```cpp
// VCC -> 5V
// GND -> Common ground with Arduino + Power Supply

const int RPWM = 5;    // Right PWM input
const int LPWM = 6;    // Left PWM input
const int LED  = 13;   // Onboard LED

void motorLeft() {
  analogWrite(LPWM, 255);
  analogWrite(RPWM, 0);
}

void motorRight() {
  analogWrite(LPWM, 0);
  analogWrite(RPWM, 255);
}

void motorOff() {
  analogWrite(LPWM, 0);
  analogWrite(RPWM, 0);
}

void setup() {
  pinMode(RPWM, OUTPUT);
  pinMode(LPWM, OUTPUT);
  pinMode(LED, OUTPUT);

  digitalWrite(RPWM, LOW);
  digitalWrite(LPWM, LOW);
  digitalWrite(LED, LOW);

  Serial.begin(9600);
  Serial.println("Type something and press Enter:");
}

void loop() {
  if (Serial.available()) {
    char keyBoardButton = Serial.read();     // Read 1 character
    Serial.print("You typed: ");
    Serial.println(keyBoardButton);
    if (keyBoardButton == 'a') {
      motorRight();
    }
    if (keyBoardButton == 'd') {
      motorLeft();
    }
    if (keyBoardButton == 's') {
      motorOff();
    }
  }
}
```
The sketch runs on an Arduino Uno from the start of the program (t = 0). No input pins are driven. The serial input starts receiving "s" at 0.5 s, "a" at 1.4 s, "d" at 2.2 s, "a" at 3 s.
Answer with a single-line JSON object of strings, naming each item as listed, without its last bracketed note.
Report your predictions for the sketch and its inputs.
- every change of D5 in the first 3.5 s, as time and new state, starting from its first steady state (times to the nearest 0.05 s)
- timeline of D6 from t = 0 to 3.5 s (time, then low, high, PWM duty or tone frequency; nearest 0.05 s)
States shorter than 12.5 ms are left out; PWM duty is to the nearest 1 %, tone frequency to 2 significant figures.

{"every change of D5 in the first 3.5 s, as time and new state, starting from its first steady state": "0 s low; 1.4 s high; 2.2 s low; 3 s high", "timeline of D6 from t = 0 to 3.5 s": "0 s low; 2.2 s high; 3 s low"}
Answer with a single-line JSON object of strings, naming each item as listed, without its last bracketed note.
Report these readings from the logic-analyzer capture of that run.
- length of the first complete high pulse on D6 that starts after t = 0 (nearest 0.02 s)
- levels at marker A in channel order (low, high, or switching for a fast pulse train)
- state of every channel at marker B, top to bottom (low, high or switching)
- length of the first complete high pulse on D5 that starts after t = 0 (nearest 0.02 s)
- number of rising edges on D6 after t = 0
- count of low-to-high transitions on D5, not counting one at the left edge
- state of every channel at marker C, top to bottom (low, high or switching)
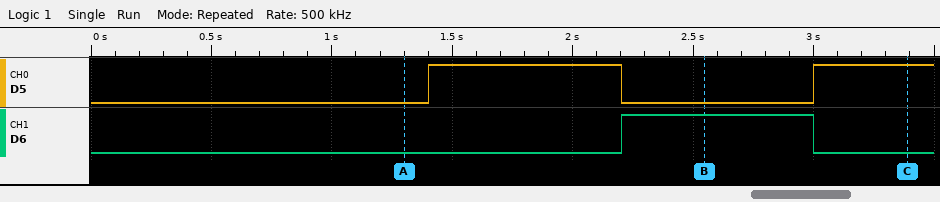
{"length of the first complete high pulse on D6 that starts after t = 0": "0.80 s", "levels at marker A in channel order": "D5 low, D6 low", "state of every channel at marker B, top to bottom": "D5 low, D6 high", "length of the first complete high pulse on D5 that starts after t = 0": "0.80 s", "number of rising edges on D6 after t = 0": "1", "count of low-to-high transitions on D5, not counting one at the left edge": "2", "state of every channel at marker C, top to bottom": "D5 high, D6 low"}
